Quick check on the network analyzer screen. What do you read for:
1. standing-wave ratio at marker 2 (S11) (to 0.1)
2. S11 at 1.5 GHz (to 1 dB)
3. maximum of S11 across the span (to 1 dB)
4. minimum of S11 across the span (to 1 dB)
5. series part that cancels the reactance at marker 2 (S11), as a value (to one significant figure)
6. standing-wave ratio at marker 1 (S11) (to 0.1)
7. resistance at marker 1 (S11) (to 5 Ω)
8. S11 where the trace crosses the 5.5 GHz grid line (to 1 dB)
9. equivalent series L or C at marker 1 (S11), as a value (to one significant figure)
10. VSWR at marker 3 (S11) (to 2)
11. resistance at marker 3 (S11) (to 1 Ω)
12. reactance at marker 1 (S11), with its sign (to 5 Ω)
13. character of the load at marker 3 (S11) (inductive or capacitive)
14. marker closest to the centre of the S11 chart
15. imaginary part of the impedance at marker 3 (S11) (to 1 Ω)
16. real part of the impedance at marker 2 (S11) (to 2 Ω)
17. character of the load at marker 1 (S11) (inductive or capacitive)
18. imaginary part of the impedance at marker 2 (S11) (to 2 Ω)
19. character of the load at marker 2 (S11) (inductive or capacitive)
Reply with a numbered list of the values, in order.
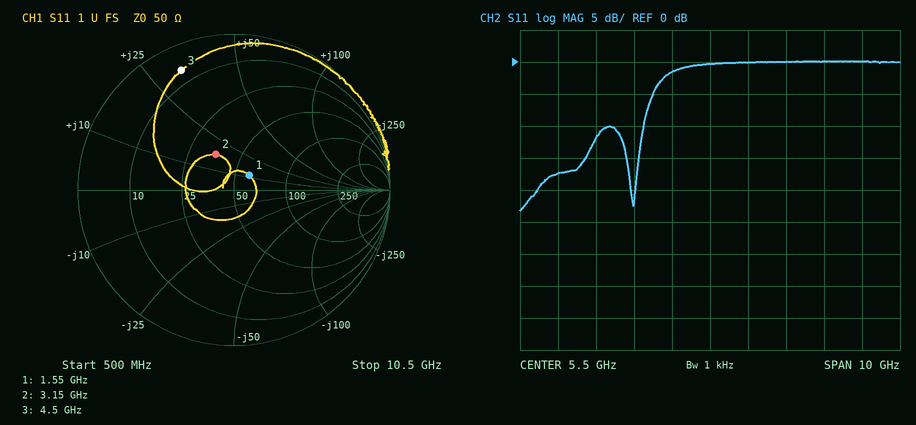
1. 1.7
2. -17 dB
3. 0 dB
4. -23 dB
5. 3 pF
6. 1.3
7. 60 Ω
8. 0 dB
9. 1 nH
10. 12
11. 6 Ω
12. +10 Ω
13. inductive
14. marker 1
15. +32 Ω
16. 36 Ω
17. inductive
18. +18 Ω
19. inductive
